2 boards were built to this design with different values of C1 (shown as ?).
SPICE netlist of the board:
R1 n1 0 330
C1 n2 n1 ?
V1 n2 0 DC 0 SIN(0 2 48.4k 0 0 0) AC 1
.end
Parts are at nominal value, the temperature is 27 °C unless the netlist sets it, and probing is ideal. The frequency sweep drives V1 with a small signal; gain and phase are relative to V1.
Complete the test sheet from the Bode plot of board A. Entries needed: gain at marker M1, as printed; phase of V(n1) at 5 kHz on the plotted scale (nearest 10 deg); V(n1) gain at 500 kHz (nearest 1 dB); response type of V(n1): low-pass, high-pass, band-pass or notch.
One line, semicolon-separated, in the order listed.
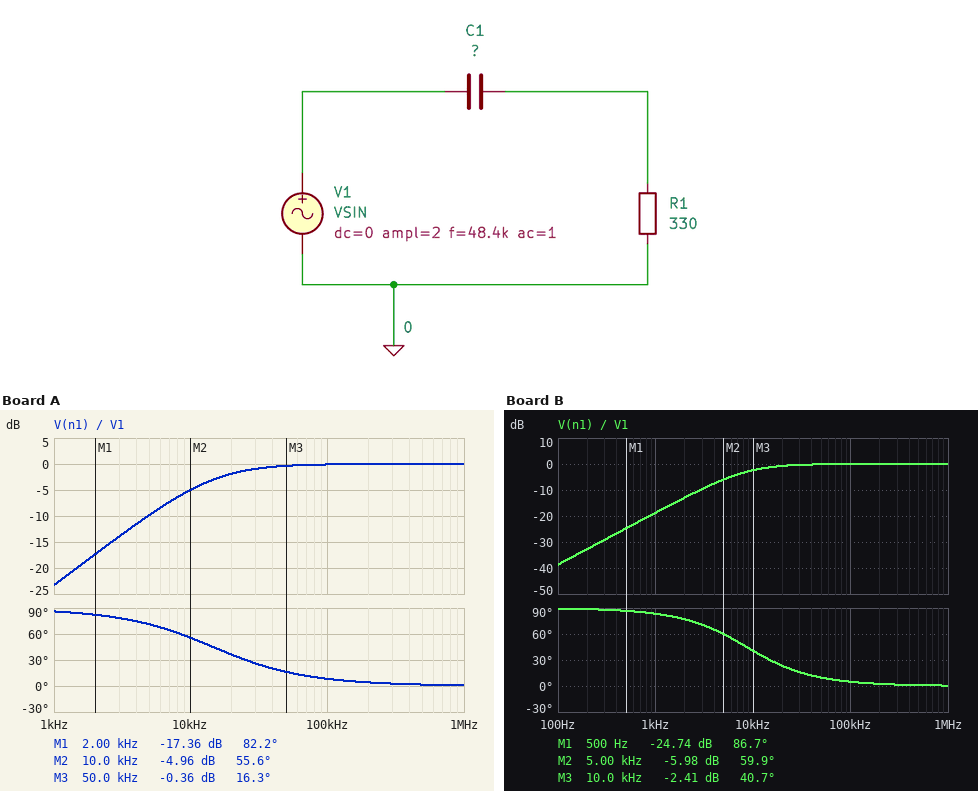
-17.36 dB; 70 deg; 0 dB; high-pass
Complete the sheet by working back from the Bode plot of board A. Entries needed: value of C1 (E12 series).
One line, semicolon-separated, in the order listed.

33 nF
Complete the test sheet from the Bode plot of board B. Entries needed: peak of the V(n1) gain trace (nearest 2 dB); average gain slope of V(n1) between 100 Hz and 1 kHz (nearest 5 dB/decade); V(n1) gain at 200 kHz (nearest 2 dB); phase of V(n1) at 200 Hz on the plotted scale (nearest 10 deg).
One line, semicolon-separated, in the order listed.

0 dB; 20 dB/decade; 0 dB; 90 deg
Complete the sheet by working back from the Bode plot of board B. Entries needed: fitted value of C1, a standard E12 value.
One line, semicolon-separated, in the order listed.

56 nF
